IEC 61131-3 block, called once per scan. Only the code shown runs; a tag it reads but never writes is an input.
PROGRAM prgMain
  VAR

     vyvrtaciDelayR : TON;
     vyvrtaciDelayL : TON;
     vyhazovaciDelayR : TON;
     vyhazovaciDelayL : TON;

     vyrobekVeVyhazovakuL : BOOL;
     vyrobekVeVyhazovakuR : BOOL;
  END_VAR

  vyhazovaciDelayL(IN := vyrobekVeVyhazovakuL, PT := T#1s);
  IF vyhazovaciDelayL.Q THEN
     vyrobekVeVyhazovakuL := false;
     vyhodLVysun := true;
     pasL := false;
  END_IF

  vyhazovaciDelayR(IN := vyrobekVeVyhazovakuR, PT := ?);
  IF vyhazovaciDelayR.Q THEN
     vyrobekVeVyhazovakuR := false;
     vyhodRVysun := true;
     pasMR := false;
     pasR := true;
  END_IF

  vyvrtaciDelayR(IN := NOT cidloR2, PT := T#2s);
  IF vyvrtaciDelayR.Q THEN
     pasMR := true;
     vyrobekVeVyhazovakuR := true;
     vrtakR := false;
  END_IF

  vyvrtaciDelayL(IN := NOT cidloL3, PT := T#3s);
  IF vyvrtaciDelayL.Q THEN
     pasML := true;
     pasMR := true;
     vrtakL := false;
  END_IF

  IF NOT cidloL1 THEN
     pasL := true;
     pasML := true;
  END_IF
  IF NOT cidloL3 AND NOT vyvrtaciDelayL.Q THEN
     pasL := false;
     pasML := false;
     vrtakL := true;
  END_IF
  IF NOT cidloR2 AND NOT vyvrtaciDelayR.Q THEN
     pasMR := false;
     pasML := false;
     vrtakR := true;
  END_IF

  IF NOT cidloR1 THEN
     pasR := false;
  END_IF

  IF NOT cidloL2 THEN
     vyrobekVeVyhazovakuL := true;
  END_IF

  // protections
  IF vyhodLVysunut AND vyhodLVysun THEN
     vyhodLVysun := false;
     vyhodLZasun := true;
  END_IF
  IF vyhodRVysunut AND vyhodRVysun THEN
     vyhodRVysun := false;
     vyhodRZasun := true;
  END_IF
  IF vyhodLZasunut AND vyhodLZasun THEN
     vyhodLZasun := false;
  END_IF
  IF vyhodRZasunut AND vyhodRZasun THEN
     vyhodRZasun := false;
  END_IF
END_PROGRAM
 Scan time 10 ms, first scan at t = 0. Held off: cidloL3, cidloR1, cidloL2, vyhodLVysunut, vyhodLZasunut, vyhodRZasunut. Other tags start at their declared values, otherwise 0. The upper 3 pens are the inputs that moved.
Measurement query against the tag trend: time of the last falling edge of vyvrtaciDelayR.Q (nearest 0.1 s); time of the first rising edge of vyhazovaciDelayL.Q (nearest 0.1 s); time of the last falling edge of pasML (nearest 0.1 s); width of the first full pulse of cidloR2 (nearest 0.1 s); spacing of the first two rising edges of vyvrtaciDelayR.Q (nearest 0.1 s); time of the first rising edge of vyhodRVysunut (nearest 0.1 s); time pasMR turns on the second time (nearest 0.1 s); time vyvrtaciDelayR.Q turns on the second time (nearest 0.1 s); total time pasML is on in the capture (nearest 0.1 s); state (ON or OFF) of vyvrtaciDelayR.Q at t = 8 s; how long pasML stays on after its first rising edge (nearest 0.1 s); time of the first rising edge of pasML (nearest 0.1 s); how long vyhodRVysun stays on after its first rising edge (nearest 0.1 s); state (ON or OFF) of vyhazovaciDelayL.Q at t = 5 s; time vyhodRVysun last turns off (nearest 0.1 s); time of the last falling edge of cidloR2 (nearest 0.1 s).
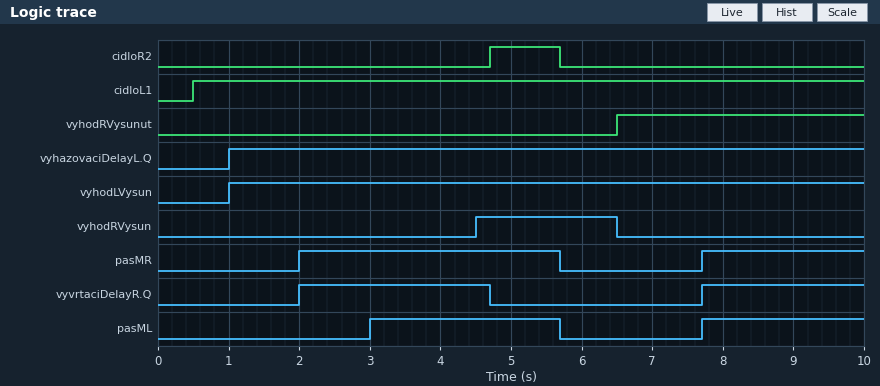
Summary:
4.7 s
1.0 s
5.7 s
1.0 s
5.7 s
6.5 s
7.7 s
7.7 s
5.0 s
ON
2.7 s
3.0 s
2.0 s
ON
6.5 s
5.7 s
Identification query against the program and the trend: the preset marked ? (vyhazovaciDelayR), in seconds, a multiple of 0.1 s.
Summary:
2.5 s
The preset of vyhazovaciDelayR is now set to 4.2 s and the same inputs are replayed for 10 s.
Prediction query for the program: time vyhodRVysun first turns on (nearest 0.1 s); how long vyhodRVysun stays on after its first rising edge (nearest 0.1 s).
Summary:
6.2 s
0.3 s
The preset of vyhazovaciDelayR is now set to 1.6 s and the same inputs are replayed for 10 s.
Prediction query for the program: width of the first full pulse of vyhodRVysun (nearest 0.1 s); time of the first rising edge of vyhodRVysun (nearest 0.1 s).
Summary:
2.9 s
3.6 s
